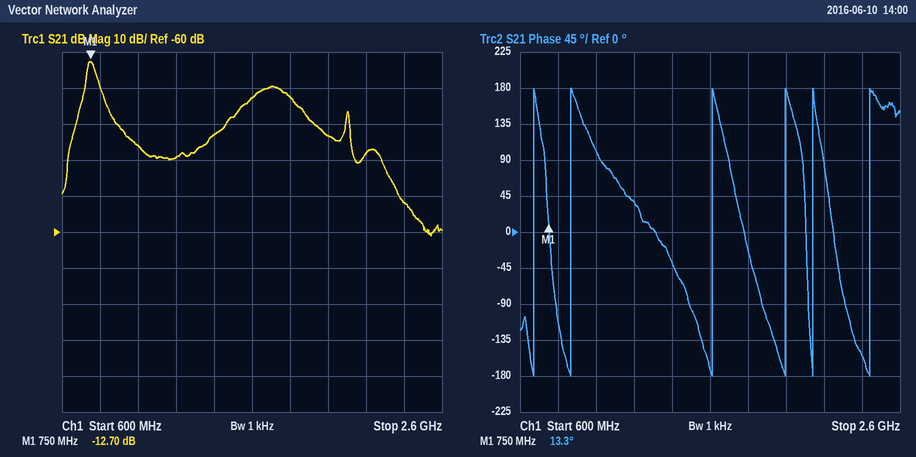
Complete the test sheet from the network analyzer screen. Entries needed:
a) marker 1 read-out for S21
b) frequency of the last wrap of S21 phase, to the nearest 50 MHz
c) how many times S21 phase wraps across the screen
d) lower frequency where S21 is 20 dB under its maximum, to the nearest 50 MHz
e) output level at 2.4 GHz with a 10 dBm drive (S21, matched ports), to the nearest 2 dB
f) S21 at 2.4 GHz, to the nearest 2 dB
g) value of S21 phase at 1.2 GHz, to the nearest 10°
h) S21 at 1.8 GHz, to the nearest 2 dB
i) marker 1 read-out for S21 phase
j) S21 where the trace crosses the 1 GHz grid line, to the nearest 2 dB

-12.70 dB
2.45 GHz
6
650 MHz
-42 dBm
-52 dB
40°
-22 dB
13.3°
-36 dB
